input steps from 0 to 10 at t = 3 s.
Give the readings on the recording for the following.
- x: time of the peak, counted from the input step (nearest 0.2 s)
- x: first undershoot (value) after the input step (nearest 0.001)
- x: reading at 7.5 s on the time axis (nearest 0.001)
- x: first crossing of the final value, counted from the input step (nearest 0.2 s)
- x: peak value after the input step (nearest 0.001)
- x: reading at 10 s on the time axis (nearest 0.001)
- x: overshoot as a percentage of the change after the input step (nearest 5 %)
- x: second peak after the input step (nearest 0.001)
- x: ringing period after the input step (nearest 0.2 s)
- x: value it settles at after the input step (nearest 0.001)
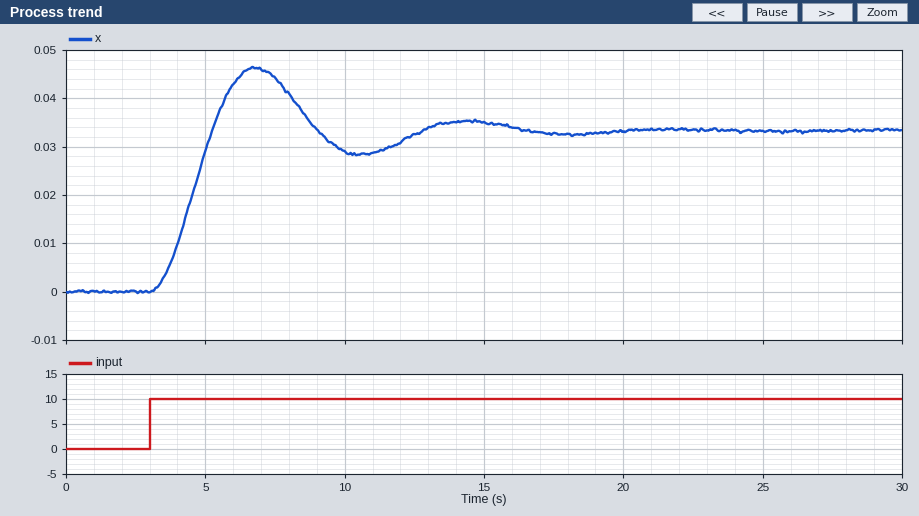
3.8 s
0.028
0.044
2.2 s
0.046
0.029
40 %
0.035
7.6 s
0.033
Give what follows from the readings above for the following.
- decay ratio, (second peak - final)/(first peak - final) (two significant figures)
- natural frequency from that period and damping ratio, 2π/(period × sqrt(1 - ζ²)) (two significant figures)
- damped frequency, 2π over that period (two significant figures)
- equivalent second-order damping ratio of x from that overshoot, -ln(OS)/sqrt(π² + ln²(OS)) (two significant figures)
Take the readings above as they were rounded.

0.15
0.86 rad/s
0.83 rad/s
0.28
